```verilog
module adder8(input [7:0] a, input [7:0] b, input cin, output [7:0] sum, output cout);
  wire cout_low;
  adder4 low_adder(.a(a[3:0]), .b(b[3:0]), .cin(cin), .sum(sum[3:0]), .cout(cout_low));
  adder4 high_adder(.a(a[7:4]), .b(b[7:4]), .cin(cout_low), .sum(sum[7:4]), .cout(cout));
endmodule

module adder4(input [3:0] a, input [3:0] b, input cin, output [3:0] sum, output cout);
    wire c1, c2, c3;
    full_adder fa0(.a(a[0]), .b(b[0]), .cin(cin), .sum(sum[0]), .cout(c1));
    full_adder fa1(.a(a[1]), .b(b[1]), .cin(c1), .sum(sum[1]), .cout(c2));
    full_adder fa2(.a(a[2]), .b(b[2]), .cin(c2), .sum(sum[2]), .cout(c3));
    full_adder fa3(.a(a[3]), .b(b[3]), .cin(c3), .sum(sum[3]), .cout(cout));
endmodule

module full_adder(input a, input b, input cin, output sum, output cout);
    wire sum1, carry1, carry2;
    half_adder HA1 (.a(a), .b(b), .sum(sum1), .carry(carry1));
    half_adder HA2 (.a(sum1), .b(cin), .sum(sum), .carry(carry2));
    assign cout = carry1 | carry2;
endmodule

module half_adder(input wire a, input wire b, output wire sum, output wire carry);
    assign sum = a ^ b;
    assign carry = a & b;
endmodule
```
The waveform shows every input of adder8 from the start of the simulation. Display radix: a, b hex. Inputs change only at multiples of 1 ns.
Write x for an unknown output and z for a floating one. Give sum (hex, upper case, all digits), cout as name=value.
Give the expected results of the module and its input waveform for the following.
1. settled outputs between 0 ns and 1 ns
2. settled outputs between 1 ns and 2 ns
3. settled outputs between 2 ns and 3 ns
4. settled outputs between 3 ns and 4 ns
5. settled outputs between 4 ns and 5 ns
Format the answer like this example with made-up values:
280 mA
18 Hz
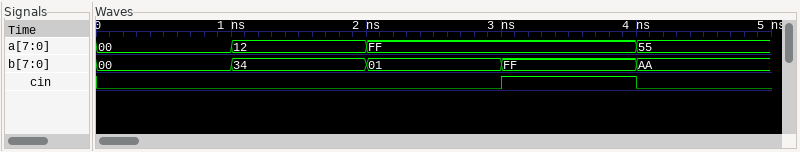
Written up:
sum=00, cout=0
sum=46, cout=0
sum=00, cout=1
sum=FF, cout=1
sum=FF, cout=0
